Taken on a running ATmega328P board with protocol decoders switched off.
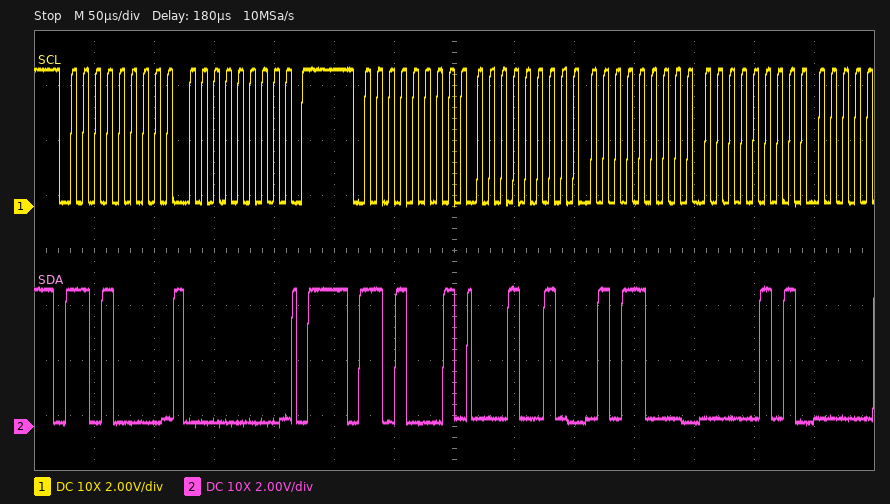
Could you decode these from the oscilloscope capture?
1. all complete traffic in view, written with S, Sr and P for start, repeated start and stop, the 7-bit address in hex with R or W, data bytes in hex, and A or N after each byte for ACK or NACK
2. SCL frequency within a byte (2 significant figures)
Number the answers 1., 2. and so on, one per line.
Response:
1. S 68W A 00 A P S 68R A 12 A 58 A 05 A
2. 100 kHz
